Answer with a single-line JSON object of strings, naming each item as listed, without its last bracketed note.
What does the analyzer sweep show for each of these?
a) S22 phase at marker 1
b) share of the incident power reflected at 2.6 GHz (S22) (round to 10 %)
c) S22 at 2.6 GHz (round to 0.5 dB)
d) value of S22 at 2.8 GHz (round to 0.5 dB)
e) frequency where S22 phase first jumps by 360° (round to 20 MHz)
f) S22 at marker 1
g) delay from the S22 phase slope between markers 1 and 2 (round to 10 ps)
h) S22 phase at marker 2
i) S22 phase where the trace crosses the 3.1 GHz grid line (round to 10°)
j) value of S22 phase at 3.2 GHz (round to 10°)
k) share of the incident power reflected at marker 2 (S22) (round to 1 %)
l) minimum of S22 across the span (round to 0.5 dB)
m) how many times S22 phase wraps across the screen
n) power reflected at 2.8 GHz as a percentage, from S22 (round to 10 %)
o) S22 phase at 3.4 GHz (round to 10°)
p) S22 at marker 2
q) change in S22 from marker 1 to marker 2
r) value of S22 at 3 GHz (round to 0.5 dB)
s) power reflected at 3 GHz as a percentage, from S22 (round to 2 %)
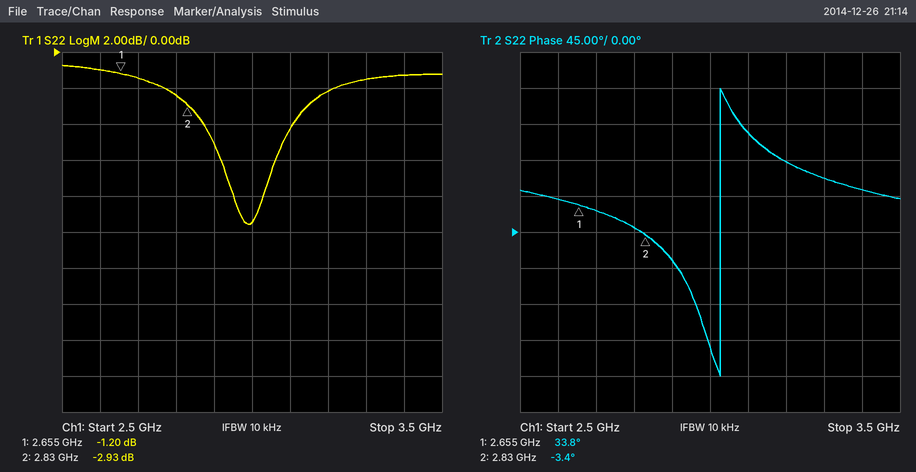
{"S22 phase at marker 1": "33.8°", "share of the incident power reflected at 2.6 GHz (S22)": "80 %", "S22 at 2.6 GHz": "-1.0 dB", "value of S22 at 2.8 GHz": "-2.5 dB", "frequency where S22 phase first jumps by 360°": "3.02 GHz", "S22 at marker 1": "-1.20 dB", "delay from the S22 phase slope between markers 1 and 2": "590 ps", "S22 phase at marker 2": "-3.4°", "S22 phase where the trace crosses the 3.1 GHz grid line": "120°", "value of S22 phase at 3.2 GHz": "90°", "share of the incident power reflected at marker 2 (S22)": "51 %", "minimum of S22 across the span": "-9.5 dB", "how many times S22 phase wraps across the screen": "1", "power reflected at 2.8 GHz as a percentage, from S22": "60 %", "S22 phase at 3.4 GHz": "50°", "S22 at marker 2": "-2.93 dB", "change in S22 from marker 1 to marker 2": "-1.73 dB", "value of S22 at 3 GHz": "-9.5 dB", "power reflected at 3 GHz as a percentage, from S22": "12 %"}
